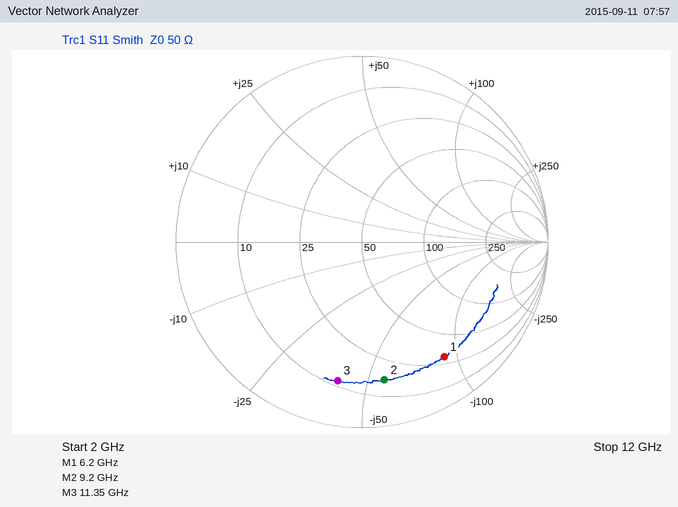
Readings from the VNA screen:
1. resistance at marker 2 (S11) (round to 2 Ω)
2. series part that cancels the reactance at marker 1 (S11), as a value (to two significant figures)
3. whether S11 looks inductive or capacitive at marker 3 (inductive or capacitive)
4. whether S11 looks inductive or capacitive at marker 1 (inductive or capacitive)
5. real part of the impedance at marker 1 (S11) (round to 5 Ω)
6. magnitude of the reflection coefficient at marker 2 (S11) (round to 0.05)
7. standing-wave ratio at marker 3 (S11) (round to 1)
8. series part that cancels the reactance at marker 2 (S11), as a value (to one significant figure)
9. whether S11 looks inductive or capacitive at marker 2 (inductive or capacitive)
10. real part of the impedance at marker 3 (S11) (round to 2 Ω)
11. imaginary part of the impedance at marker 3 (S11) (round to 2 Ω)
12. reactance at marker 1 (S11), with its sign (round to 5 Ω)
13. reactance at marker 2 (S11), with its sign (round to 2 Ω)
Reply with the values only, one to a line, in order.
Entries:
16 Ω
2.3 nH
capacitive
capacitive
30 Ω
0.75
7
1.0 nH
capacitive
12 Ω
-40 Ω
-90 Ω
-56 Ω
